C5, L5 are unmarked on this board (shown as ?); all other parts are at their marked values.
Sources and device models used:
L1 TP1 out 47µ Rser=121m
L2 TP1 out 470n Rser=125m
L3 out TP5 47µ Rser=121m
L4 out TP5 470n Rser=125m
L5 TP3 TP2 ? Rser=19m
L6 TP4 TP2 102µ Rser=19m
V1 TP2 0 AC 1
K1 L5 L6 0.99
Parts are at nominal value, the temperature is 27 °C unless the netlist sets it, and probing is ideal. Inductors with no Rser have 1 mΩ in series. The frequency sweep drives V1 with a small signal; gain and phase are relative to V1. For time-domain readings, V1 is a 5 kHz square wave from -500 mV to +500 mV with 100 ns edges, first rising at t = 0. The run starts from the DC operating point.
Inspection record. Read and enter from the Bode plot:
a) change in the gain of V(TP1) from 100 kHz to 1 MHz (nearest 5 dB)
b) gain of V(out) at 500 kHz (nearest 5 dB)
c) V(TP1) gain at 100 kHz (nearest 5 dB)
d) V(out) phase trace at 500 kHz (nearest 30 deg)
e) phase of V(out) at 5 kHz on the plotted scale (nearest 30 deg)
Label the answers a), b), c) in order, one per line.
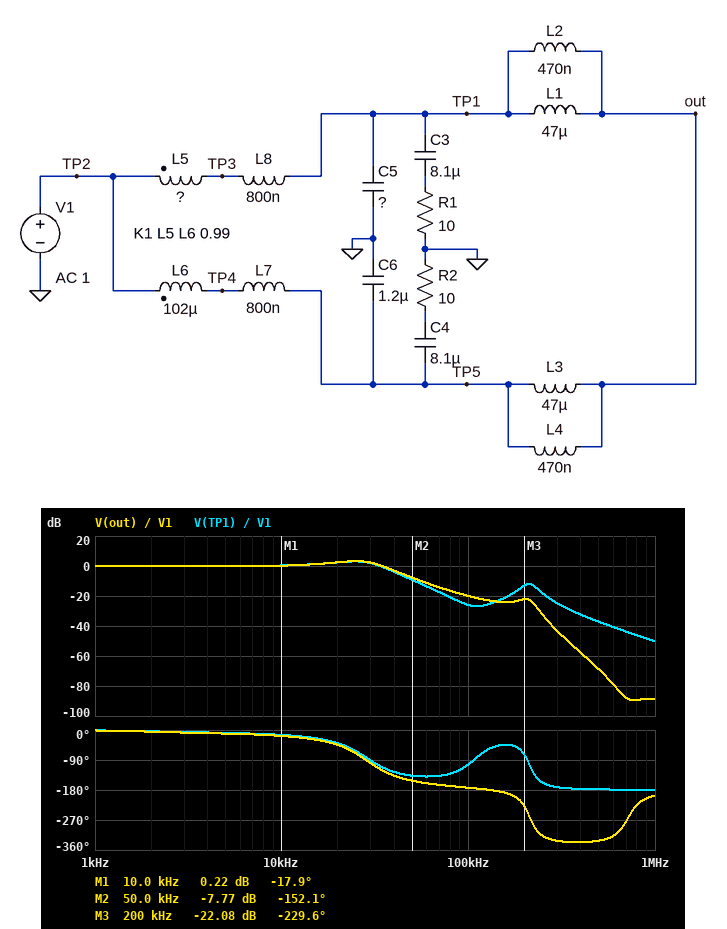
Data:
a) -25 dB
b) -70 dB
c) -25 dB
d) -330 deg
e) 0 deg
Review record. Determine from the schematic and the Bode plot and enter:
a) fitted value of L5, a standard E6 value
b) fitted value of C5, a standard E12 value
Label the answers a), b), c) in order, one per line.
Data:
a) 33 µH
b) 2.2 µF
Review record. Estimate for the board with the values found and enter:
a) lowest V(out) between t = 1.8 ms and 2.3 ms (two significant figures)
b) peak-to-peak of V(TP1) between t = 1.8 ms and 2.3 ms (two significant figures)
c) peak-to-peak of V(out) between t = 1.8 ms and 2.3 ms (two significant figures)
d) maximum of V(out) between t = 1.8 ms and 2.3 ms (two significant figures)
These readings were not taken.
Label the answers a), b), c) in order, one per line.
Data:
a) -740 mV
b) 1.5 V
c) 1.5 V
d) 740 mV
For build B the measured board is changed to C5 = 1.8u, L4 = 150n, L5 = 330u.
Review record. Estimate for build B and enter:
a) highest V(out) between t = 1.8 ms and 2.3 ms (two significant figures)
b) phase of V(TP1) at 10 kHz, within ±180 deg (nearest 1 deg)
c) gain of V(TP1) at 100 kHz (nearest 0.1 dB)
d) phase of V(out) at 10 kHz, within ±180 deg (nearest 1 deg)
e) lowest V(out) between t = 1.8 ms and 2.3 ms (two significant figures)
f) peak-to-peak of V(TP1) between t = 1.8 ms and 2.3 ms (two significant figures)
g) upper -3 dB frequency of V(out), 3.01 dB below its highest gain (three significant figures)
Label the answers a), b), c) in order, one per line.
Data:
a) 660 mV
b) -26 deg
c) -21.6 dB
d) -23 deg
e) -660 mV
f) 1.3 V
g) 28.3 kHz
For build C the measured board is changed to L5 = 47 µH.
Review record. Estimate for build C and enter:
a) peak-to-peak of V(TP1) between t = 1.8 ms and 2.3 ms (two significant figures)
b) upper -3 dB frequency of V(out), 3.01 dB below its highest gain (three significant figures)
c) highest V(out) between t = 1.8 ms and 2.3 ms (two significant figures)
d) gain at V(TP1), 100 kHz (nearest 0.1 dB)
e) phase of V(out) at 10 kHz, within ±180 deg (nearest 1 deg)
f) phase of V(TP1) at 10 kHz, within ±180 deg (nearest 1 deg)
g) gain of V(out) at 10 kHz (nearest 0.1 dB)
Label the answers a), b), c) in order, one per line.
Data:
a) 1.3 V
b) 24.9 kHz
c) 630 mV
d) -31.0 dB
e) -33 deg
f) -29 deg
g) 0.5 dB
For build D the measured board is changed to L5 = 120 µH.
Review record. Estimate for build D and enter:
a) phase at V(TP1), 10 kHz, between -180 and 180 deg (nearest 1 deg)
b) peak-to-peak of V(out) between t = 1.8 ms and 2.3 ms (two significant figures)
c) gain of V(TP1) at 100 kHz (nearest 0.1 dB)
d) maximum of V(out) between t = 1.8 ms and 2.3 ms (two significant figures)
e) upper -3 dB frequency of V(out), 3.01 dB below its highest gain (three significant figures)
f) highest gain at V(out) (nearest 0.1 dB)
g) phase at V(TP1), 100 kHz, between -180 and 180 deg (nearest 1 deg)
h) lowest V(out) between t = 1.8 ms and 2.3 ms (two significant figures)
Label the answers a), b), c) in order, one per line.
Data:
a) -114 deg
b) 1.5 V
c) -36.2 dB
d) 770 mV
e) 7.79 kHz
f) 2.6 dB
g) 169 deg
h) -770 mV
